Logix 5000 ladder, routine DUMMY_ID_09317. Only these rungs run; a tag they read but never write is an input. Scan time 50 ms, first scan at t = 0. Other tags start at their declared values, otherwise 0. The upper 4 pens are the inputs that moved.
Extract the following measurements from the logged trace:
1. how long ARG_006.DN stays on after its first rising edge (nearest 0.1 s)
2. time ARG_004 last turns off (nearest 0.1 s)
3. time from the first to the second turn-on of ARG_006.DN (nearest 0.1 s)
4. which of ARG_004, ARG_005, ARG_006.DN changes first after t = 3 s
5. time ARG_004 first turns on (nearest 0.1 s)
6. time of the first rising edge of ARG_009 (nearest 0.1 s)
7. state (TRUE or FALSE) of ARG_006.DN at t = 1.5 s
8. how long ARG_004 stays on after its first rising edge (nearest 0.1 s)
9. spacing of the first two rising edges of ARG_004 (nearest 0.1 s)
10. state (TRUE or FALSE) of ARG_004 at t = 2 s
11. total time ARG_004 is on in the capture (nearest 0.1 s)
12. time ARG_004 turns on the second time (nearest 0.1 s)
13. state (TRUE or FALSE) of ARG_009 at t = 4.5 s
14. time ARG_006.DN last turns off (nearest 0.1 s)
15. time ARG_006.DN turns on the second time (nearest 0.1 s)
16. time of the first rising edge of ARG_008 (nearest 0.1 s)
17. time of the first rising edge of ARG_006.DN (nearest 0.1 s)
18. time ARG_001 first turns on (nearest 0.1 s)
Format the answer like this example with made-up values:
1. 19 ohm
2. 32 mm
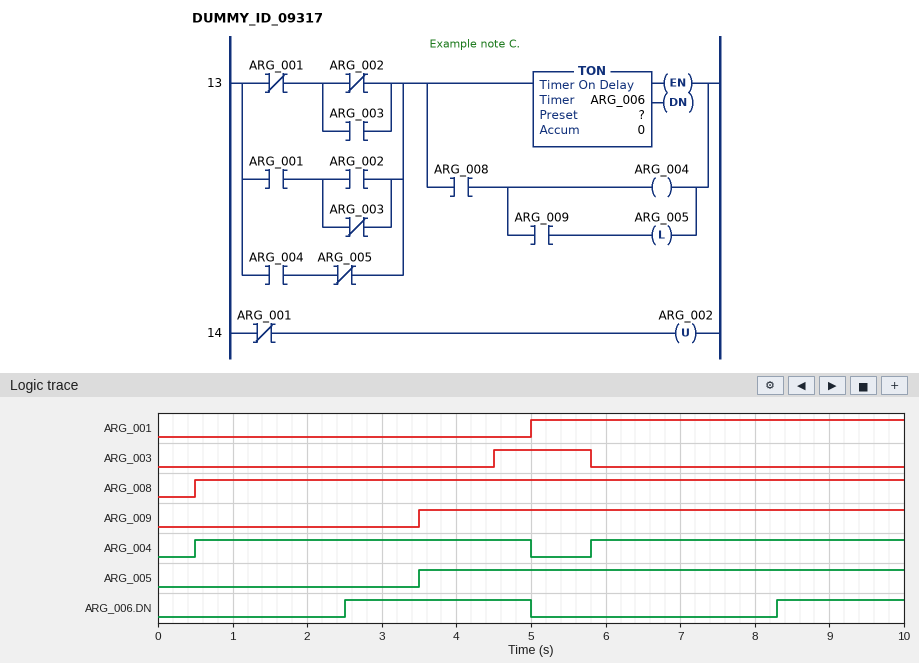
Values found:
1. 2.5 s
2. 5.0 s
3. 5.8 s
4. ARG_005
5. 0.5 s
6. 3.5 s
7. FALSE
8. 4.5 s
9. 5.3 s
10. TRUE
11. 8.7 s
12. 5.8 s
13. TRUE
14. 5.0 s
15. 8.3 s
16. 0.5 s
17. 2.5 s
18. 5.0 s
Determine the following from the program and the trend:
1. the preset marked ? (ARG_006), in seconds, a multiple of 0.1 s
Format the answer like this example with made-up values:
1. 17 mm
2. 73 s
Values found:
1. 2.5 s
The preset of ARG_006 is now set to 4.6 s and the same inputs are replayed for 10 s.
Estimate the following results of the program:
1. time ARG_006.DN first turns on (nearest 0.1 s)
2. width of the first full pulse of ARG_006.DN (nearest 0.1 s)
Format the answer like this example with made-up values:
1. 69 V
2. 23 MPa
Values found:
1. 4.6 s
2. 0.4 s
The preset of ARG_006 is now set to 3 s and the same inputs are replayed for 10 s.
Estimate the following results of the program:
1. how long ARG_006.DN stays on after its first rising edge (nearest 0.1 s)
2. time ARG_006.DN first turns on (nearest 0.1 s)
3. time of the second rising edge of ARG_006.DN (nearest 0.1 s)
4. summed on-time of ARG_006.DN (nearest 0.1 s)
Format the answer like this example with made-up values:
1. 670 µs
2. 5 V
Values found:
1. 2.0 s
2. 3.0 s
3. 8.8 s
4. 3.2 s
